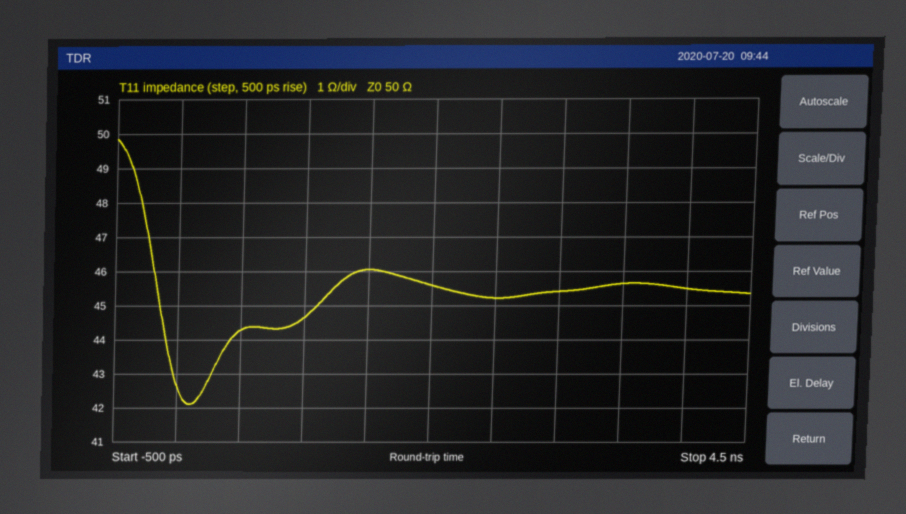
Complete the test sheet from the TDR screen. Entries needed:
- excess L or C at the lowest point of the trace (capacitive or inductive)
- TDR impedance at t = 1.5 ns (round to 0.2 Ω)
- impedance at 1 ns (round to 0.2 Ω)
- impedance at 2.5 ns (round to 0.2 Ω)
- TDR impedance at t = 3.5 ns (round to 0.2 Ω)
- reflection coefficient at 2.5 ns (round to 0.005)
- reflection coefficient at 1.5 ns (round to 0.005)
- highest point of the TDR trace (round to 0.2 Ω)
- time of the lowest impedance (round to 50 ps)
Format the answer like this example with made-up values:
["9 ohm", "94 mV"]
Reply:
["capacitive", "46.0 Ω", "44.6 Ω", "45.2 Ω", "45.6 Ω", "-0.050", "-0.040", "49.8 Ω", "100 ps"]
